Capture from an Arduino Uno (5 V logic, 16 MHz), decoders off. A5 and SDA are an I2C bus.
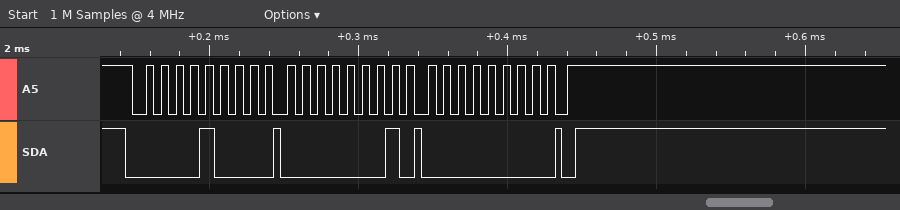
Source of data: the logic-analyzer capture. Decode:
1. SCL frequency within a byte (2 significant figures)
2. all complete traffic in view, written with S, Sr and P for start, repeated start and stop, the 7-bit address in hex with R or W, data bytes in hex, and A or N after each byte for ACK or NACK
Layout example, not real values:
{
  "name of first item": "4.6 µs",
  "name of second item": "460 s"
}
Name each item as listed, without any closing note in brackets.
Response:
{
  "SCL frequency within a byte": "100 kHz",
  "all complete traffic in view, written with S, Sr and P for start, repeated start and stop, the 7-bit address in hex with R or W, data bytes in hex, and A or N after each byte for ACK or NACK": "S 04W A 01 A 00 A P"
}
